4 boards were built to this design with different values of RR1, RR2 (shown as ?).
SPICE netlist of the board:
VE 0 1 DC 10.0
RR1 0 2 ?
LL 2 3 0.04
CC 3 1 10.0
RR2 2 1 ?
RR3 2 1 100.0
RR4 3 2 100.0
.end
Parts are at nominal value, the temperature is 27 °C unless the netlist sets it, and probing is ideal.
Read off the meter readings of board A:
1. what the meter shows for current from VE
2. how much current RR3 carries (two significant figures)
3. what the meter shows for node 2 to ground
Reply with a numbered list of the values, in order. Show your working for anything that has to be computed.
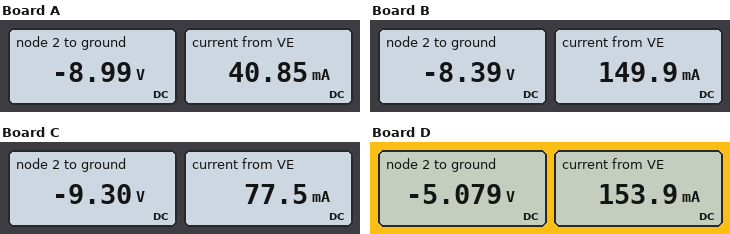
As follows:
1. 40.85 mA
2. (-8.99 V - (-10 V)) / 100 Ω = 10 mA
3. -8.99 V
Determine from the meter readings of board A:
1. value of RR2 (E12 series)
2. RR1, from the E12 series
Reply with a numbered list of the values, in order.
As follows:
1. 33 Ω
2. 220 Ω
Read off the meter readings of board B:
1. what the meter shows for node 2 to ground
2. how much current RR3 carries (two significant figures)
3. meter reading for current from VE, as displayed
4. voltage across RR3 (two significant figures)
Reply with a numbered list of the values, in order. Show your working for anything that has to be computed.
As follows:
1. -8.39 V
2. (-8.39 V - (-10 V)) / 100 Ω = 16 mA
3. 149.9 mA
4. -8.39 V - (-10 V) = 1.6 V
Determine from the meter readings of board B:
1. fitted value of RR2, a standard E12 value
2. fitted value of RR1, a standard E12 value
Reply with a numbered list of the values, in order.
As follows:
1. 12 Ω
2. 56 Ω
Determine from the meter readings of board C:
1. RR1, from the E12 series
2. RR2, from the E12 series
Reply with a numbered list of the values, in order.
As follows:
1. 120 Ω
2. 10 Ω
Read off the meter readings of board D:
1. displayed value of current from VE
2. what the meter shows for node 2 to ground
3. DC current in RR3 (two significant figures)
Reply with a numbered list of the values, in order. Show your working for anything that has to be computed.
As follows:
1. 153.9 mA
2. -5.079 V
3. (-5.079 V - (-10 V)) / 100 Ω = 49 mA
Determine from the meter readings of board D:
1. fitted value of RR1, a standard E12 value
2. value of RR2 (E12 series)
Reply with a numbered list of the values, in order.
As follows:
1. 33 Ω
2. 47 Ω
